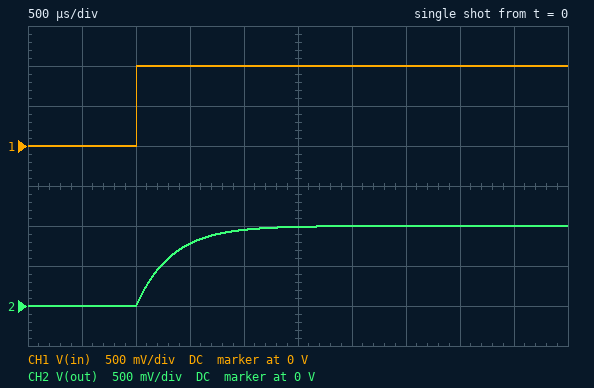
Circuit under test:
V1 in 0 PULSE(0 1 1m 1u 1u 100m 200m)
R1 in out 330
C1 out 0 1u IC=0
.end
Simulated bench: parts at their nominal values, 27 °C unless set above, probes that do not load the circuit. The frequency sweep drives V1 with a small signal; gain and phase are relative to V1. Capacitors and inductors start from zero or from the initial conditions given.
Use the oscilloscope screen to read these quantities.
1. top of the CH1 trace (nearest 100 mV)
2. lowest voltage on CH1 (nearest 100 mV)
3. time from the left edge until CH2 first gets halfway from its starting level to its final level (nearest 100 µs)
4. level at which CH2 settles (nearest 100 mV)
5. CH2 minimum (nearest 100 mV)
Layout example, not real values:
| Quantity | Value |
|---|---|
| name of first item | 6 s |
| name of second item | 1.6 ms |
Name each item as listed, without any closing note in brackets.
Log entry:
| Quantity | Value |
|---|---|
| top of the CH1 trace | 1.0 V |
| lowest voltage on CH1 | 0 V |
| time from the left edge until CH2 first gets halfway from its starting level to its final level | 1.2 ms |
| level at which CH2 settles | 1.0 V |
| CH2 minimum | 0 V |
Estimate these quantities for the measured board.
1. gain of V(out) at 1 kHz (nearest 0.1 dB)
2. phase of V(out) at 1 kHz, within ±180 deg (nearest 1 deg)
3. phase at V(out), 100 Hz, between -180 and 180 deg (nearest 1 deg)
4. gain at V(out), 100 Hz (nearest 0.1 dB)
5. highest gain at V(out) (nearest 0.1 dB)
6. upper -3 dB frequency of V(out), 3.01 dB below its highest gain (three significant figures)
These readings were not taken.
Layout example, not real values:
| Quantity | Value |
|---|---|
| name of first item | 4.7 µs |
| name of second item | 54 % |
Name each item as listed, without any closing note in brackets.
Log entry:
| Quantity | Value |
|---|---|
| gain of V(out) at 1 kHz | -7.2 dB |
| phase of V(out) at 1 kHz, within ±180 deg | -64 deg |
| phase at V(out), 100 Hz, between -180 and 180 deg | -12 deg |
| gain at V(out), 100 Hz | -0.2 dB |
| highest gain at V(out) | 0 dB |
| upper -3 dB frequency of V(out), 3.01 dB below its highest gain | 482 Hz |
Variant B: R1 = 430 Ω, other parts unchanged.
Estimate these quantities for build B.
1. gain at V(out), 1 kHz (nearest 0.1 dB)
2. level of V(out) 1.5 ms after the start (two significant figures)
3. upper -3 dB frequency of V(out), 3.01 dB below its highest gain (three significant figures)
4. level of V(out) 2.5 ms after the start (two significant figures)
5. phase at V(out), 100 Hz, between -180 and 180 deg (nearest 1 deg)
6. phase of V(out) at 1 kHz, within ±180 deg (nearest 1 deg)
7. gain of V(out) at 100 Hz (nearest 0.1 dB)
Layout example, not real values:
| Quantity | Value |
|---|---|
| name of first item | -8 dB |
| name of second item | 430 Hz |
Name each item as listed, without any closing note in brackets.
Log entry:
| Quantity | Value |
|---|---|
| gain at V(out), 1 kHz | -9.2 dB |
| level of V(out) 1.5 ms after the start | 690 mV |
| upper -3 dB frequency of V(out), 3.01 dB below its highest gain | 370 Hz |
| level of V(out) 2.5 ms after the start | 970 mV |
| phase at V(out), 100 Hz, between -180 and 180 deg | -15 deg |
| phase of V(out) at 1 kHz, within ±180 deg | -70 deg |
| gain of V(out) at 100 Hz | -0.3 dB |
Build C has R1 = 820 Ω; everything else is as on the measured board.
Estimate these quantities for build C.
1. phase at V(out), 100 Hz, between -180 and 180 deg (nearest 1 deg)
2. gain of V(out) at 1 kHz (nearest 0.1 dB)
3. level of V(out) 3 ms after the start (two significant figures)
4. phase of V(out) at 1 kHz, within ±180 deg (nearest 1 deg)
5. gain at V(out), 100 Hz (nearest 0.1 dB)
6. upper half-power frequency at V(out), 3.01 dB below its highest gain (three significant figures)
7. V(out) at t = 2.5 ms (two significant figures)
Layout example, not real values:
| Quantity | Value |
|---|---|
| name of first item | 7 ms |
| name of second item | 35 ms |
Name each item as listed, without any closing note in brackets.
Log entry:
| Quantity | Value |
|---|---|
| phase at V(out), 100 Hz, between -180 and 180 deg | -27 deg |
| gain of V(out) at 1 kHz | -14.4 dB |
| level of V(out) 3 ms after the start | 910 mV |
| phase of V(out) at 1 kHz, within ±180 deg | -79 deg |
| gain at V(out), 100 Hz | -1.0 dB |
| upper half-power frequency at V(out), 3.01 dB below its highest gain | 194 Hz |
| V(out) at t = 2.5 ms | 840 mV |
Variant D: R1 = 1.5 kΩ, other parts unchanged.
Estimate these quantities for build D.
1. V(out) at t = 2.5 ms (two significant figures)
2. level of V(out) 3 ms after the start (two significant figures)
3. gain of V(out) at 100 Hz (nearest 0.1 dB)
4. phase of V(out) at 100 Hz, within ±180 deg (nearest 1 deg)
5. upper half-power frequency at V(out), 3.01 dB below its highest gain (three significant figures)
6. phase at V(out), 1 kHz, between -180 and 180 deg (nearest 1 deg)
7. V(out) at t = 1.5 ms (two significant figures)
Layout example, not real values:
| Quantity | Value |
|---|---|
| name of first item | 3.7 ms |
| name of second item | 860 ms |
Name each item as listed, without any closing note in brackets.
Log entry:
| Quantity | Value |
|---|---|
| V(out) at t = 2.5 ms | 630 mV |
| level of V(out) 3 ms after the start | 740 mV |
| gain of V(out) at 100 Hz | -2.8 dB |
| phase of V(out) at 100 Hz, within ±180 deg | -43 deg |
| upper half-power frequency at V(out), 3.01 dB below its highest gain | 106 Hz |
| phase at V(out), 1 kHz, between -180 and 180 deg | -84 deg |
| V(out) at t = 1.5 ms | 280 mV |
